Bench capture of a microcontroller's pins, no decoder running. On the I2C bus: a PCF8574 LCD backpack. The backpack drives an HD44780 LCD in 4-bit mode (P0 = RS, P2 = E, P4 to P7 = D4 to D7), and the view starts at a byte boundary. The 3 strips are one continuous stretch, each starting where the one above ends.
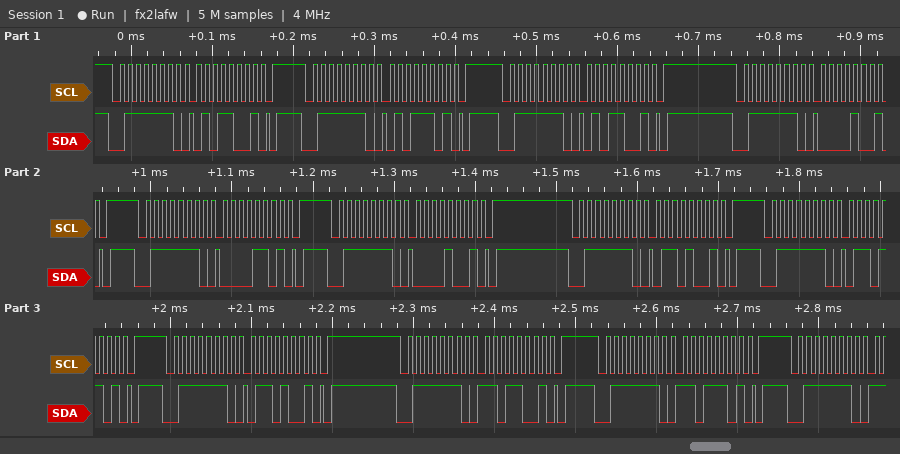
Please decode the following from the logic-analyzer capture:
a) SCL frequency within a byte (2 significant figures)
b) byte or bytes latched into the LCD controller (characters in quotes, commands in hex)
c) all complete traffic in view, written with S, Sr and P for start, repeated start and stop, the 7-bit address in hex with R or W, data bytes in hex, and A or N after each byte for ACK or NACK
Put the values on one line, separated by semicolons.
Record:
100 kHz; 'P'; S 3FW A 59 A P S 3FW A 5D A P S 3FW A 59 A P S 3FW A 09 A P S 3FW A 0D A P S 3FW A 09 A P S 3FW A 69 A P S 3FW A 6D A P S 3FW A 69 A P S 3FW A D9 A P S 3FW A DD A P S 3FW A
